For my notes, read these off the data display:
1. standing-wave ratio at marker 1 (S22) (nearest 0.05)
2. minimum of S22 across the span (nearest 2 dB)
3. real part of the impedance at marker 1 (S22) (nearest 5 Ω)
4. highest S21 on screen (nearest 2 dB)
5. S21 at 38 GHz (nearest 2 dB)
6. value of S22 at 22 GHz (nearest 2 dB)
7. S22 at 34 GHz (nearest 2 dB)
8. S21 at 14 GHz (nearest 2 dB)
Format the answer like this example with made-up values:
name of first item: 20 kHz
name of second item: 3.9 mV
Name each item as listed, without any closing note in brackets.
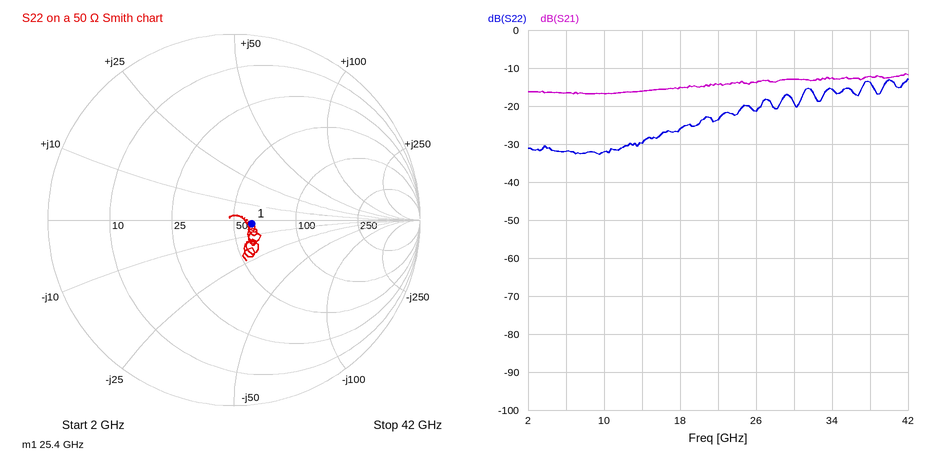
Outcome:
standing-wave ratio at marker 1 (S22): 1.20
minimum of S22 across the span: -32 dB
real part of the impedance at marker 1 (S22): 60 Ω
highest S21 on screen: -12 dB
S21 at 38 GHz: -12 dB
value of S22 at 22 GHz: -24 dB
S22 at 34 GHz: -16 dB
S21 at 14 GHz: -16 dB
